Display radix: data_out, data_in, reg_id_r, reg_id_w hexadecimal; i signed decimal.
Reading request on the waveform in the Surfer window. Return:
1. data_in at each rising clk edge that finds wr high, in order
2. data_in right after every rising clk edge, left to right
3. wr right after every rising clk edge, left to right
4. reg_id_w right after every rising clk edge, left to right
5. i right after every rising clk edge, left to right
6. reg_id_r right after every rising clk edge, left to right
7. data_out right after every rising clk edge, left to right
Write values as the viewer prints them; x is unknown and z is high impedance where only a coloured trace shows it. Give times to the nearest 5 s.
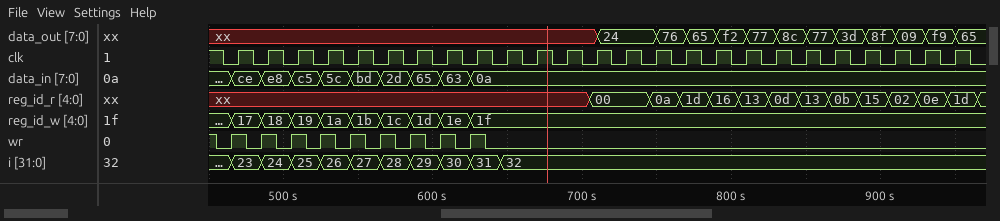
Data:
ce, e8, c5, 5c, bd, 2d, 65, 63, 0a
ce, e8, c5, 5c, bd, 2d, 65, 63, 0a, 0a, 0a, 0a, 0a, 0a, 0a, 0a, 0a, 0a, 0a, 0a, 0a, 0a, 0a, 0a, 0a
1 1 1 1 1 1 1 1 1 0 0 0 0 0 0 0 0 0 0 0 0 0 0 0 0
17, 18, 19, 1a, 1b, 1c, 1d, 1e, 1f, 1f, 1f, 1f, 1f, 1f, 1f, 1f, 1f, 1f, 1f, 1f, 1f, 1f, 1f, 1f, 1f
23, 24, 25, 26, 27, 28, 29, 30, 31, 32, 32, 32, 32, 32, 32, 32, 32, 32, 32, 32, 32, 32, 32, 32, 32
xx, xx, xx, xx, xx, xx, xx, xx, xx, xx, xx, xx, 00, 00, 0a, 1d, 16, 13, 0d, 13, 0b, 15, 02, 0e, 1d
xx, xx, xx, xx, xx, xx, xx, xx, xx, xx, xx, xx, 24, 24, 76, 65, f2, 77, 8c, 77, 3d, 8f, 09, f9, 65
